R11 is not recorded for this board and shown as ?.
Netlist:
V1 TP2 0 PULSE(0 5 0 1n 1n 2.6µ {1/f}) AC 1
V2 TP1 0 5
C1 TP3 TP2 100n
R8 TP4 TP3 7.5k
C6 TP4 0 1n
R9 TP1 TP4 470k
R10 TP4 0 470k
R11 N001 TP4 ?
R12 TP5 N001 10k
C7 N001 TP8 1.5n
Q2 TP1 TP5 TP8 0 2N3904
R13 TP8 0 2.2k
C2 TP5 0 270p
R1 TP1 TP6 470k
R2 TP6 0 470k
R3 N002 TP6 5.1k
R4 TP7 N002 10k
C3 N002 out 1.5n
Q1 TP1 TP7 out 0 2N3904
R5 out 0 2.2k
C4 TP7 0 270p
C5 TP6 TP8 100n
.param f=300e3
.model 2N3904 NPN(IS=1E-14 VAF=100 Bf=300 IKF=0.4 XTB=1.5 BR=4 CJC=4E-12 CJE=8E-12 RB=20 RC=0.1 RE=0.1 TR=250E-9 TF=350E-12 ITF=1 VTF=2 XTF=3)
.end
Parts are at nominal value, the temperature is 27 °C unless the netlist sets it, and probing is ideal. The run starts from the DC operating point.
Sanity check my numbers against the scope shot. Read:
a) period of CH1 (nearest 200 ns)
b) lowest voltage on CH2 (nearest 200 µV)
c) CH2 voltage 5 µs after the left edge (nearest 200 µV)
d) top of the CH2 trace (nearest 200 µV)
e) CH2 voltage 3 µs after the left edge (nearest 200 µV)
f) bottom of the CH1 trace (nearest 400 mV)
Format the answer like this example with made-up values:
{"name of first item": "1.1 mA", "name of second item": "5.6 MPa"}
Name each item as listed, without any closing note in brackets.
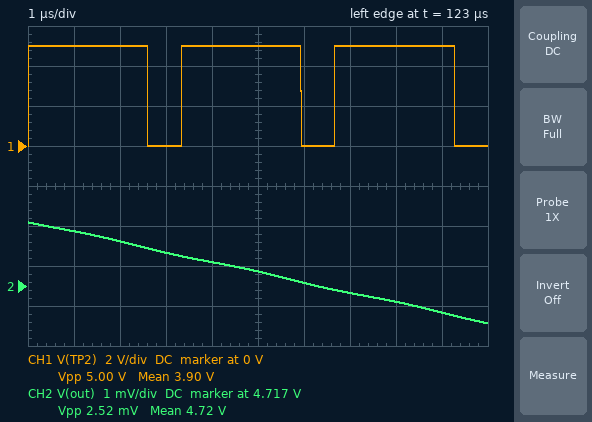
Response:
{"period of CH1": "3.4 µs", "lowest voltage on CH2": "4.7160 V", "CH2 voltage 5 µs after the left edge": "4.7174 V", "top of the CH2 trace": "4.7186 V", "CH2 voltage 3 µs after the left edge": "4.7178 V", "bottom of the CH1 trace": "0 V"}
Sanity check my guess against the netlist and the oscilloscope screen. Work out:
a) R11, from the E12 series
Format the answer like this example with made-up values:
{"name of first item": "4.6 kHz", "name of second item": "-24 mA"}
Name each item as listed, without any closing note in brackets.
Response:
{"R11, from the E12 series": "2.2 kΩ"}
